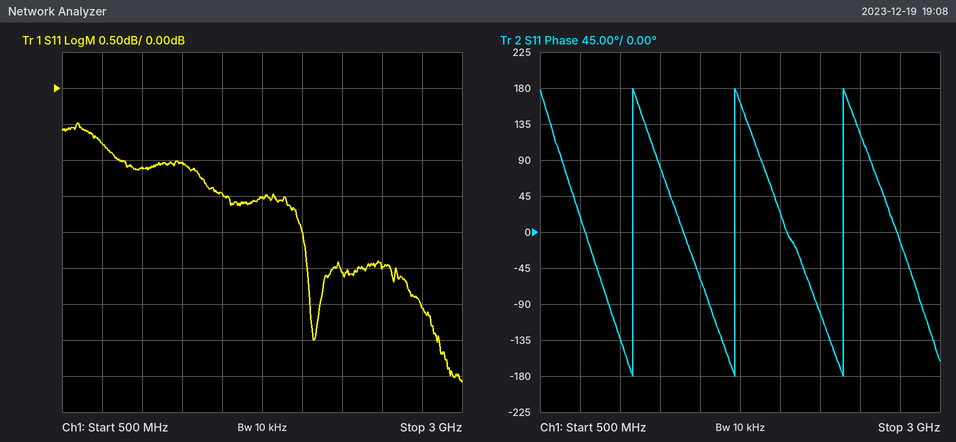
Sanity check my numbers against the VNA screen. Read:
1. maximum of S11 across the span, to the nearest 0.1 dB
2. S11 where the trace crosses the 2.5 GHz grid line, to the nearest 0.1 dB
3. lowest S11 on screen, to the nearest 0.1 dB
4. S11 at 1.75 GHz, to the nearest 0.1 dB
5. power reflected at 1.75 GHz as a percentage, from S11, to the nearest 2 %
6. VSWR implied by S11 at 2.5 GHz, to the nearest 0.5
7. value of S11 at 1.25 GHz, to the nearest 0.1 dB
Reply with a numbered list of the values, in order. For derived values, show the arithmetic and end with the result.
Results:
1. -0.5 dB
2. -2.5 dB
3. -4.1 dB
4. -1.5 dB
5. 10^(-1.5/10) ≈ 70.8 %, so 70 % to the nearest 2 %
6. |Γ| = 10^(-2.5/20) = 0.7499; VSWR = (1 + 0.7499)/(1 − 0.7499) ≈ 7.0
7. -1.0 dB
